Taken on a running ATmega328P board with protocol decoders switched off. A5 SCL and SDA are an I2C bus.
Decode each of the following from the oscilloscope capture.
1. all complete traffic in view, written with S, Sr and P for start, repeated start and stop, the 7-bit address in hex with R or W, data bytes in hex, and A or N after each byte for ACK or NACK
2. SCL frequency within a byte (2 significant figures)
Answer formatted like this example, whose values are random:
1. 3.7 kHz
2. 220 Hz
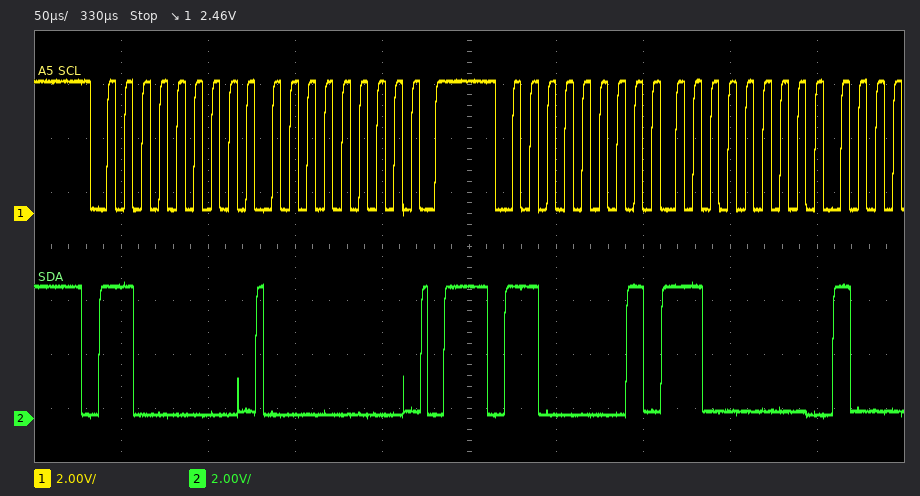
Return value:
1. S 60W A 00 A P S 60R A C0 A
2. 100 kHz
